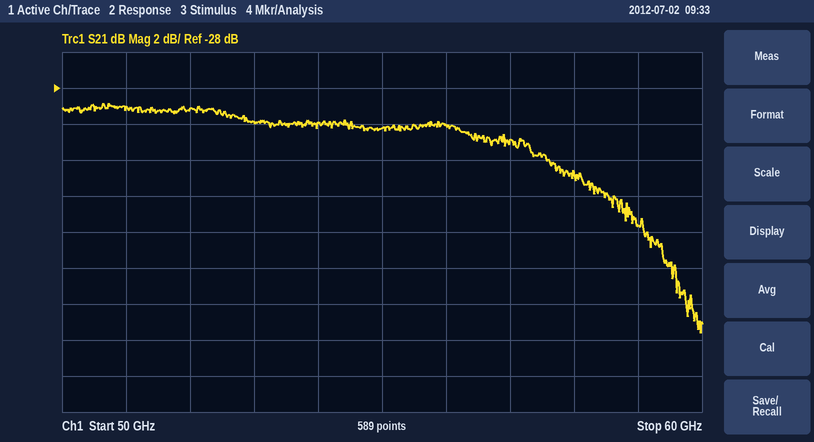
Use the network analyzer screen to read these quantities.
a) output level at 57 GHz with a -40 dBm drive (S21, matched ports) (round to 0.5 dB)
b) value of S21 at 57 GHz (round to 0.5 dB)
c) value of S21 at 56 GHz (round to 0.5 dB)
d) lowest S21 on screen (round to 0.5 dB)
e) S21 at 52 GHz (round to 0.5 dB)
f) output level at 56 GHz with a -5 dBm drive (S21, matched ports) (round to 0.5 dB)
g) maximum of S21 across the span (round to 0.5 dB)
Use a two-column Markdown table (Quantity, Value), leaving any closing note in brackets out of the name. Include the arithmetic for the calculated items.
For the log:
| Quantity | Value |
|---|---|
| output level at 57 GHz with a -40 dBm drive (S21, matched ports) | -40 dBm + (-31.0 dB) = -71.0 dBm |
| value of S21 at 57 GHz | -31.0 dB |
| value of S21 at 56 GHz | -30.0 dB |
| lowest S21 on screen | -41.5 dB |
| S21 at 52 GHz | -29.0 dB |
| output level at 56 GHz with a -5 dBm drive (S21, matched ports) | -5 dBm + (-30.0 dB) = -35.0 dBm |
| maximum of S21 across the span | -29.0 dB |
